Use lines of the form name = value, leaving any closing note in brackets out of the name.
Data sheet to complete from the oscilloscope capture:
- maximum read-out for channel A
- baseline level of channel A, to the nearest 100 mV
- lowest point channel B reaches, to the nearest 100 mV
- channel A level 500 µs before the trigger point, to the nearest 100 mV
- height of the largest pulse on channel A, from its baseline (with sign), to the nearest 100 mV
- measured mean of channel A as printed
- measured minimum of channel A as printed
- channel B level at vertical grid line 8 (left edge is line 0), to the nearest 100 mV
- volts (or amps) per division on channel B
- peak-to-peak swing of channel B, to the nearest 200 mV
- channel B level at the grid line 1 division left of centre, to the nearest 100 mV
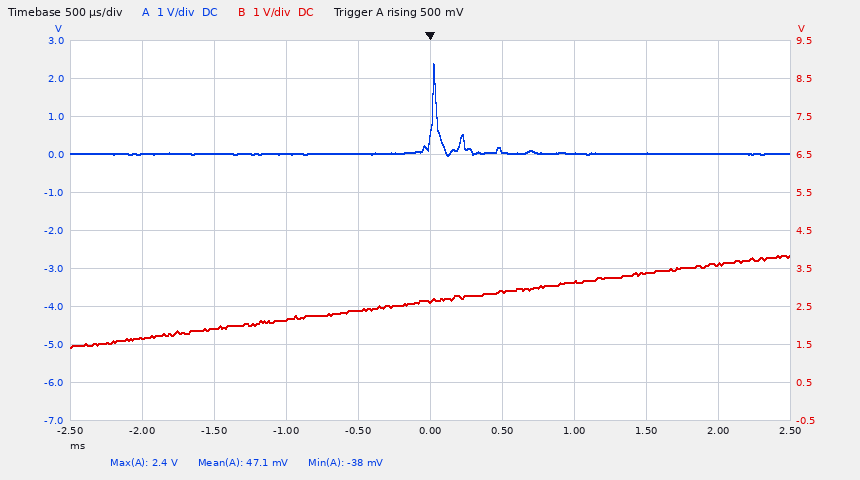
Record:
maximum read-out for channel A = 2.4 V
baseline level of channel A, to the nearest 100 mV = 0.0 V
lowest point channel B reaches, to the nearest 100 mV = 1.4 V
channel A level 500 µs before the trigger point, to the nearest 100 mV = 0.0 V
height of the largest pulse on channel A, from its baseline (with sign), to the nearest 100 mV = +2.4 V
measured mean of channel A as printed = 47.1 mV
measured minimum of channel A as printed = -38 mV
channel B level at vertical grid line 8 (left edge is line 0), to the nearest 100 mV = 3.4 V
volts (or amps) per division on channel B = 1 V
peak-to-peak swing of channel B, to the nearest 200 mV = 2.4 V
channel B level at the grid line 1 division left of centre, to the nearest 100 mV = 2.4 V
